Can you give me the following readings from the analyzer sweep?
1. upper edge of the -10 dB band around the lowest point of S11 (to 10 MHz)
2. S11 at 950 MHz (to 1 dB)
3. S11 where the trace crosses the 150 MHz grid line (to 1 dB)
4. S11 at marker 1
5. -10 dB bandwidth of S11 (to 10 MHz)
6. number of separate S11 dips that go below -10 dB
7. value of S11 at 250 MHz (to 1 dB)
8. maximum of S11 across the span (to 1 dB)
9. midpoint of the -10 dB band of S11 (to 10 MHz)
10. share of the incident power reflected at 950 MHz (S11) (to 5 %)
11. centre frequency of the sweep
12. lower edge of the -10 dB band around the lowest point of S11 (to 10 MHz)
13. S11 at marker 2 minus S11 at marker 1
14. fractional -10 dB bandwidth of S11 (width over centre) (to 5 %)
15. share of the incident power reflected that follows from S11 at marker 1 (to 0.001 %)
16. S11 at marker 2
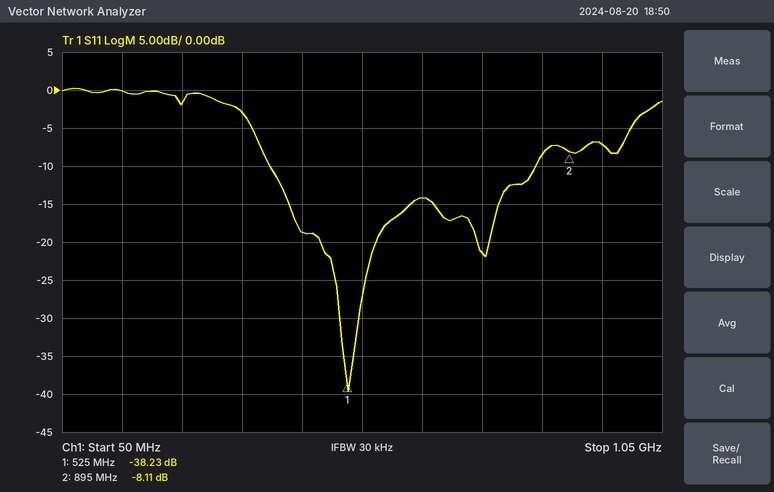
840 MHz
-7 dB
0 dB
-38.23 dB
440 MHz
2
-2 dB
0 dB
620 MHz
20 %
550 MHz
400 MHz
30.12 dB
70 %
0.015 %
-8.11 dB
